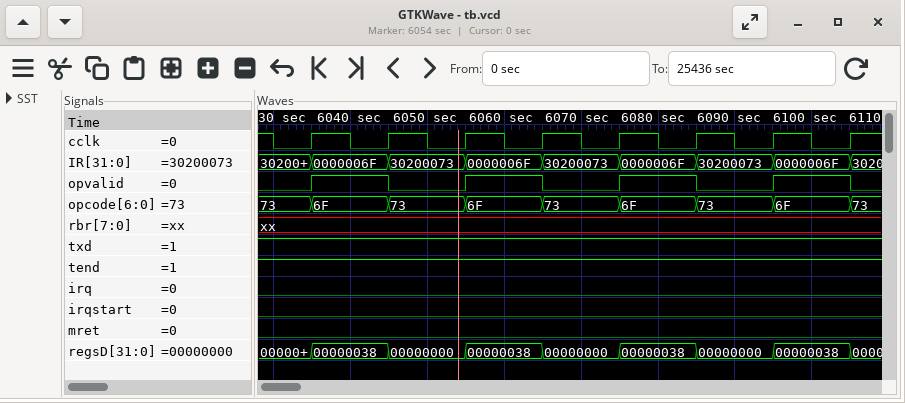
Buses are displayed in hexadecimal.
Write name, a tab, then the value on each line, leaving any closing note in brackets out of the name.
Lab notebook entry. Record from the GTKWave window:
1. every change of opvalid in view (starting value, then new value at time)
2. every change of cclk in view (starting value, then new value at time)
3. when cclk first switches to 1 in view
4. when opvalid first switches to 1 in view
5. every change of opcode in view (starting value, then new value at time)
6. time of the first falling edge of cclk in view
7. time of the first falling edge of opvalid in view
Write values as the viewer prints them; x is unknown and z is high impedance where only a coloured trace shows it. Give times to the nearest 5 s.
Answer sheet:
every change of opvalid in view	0, 1 at 6035 s, 0 at 6045 s, 1 at 6055 s, 0 at 6065 s, 1 at 6075 s, 0 at 6085 s, 1 at 6095 s, 0 at 6105 s
every change of cclk in view	1, 0 at 6030 s, 1 at 6035 s, 0 at 6040 s, 1 at 6045 s, 0 at 6050 s, 1 at 6055 s, 0 at 6060 s, 1 at 6065 s, 0 at 6070 s, 1 at 6075 s, 0 at 6080 s, 1 at 6085 s, 0 at 6090 s, 1 at 6095 s, 0 at 6100 s, 1 at 6105 s
when cclk first switches to 1 in view	6035 s
when opvalid first switches to 1 in view	6035 s
every change of opcode in view	73, 6F at 6035 s, 73 at 6045 s, 6F at 6055 s, 73 at 6065 s, 6F at 6075 s, 73 at 6085 s, 6F at 6095 s, 73 at 6105 s
time of the first falling edge of cclk in view	6030 s
time of the first falling edge of opvalid in view	6045 s
